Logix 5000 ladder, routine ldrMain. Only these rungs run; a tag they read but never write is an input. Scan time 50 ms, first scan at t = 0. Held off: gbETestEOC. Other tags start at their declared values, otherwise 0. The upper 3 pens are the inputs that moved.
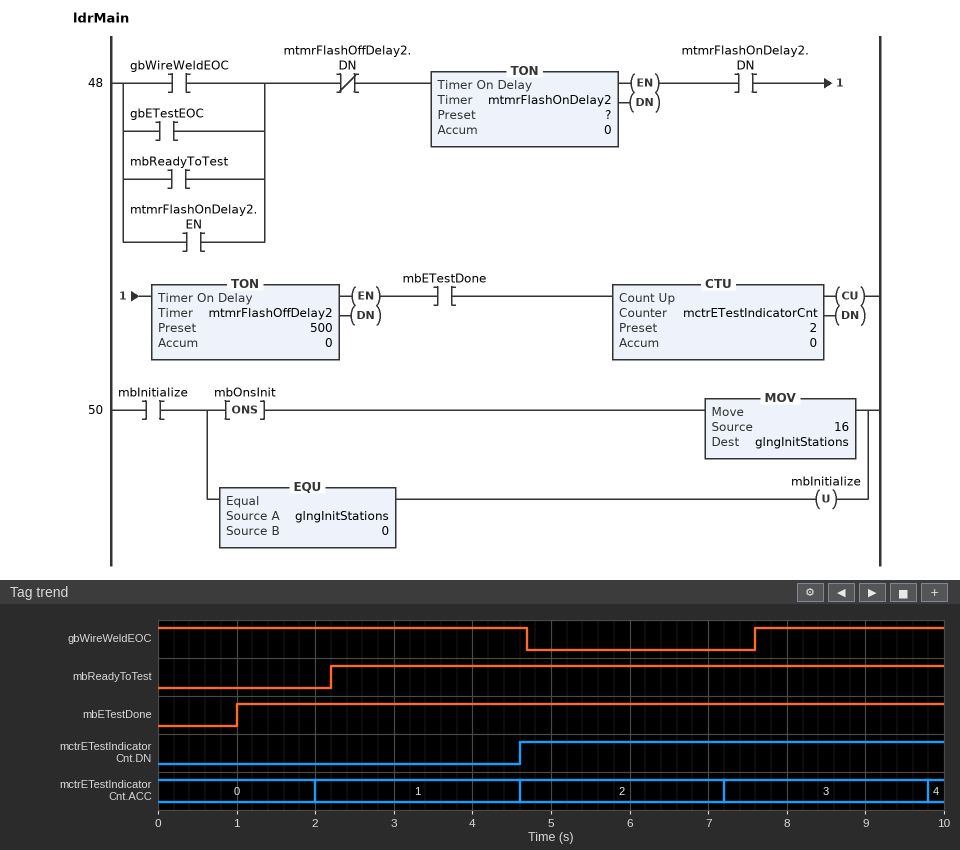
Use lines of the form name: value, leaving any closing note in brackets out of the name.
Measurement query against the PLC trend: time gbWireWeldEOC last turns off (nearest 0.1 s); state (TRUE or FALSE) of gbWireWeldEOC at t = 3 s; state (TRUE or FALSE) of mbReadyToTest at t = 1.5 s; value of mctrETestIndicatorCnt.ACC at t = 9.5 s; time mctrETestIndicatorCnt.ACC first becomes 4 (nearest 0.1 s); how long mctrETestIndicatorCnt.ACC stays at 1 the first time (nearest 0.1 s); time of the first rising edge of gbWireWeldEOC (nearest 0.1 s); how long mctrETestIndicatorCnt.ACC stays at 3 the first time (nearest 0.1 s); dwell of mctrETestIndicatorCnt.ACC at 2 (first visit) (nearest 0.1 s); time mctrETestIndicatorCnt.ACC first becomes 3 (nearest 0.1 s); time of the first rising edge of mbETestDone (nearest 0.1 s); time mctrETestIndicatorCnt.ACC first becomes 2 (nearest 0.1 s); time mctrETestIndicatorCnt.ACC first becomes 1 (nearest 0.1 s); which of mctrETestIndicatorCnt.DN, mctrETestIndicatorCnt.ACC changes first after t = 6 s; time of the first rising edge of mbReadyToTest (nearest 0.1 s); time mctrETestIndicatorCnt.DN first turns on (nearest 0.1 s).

time gbWireWeldEOC last turns off: 4.7 s
state (TRUE or FALSE) of gbWireWeldEOC at t = 3 s: TRUE
state (TRUE or FALSE) of mbReadyToTest at t = 1.5 s: FALSE
value of mctrETestIndicatorCnt.ACC at t = 9.5 s: 3
time mctrETestIndicatorCnt.ACC first becomes 4: 9.8 s
how long mctrETestIndicatorCnt.ACC stays at 1 the first time: 2.6 s
time of the first rising edge of gbWireWeldEOC: 7.6 s
how long mctrETestIndicatorCnt.ACC stays at 3 the first time: 2.6 s
dwell of mctrETestIndicatorCnt.ACC at 2 (first visit): 2.6 s
time mctrETestIndicatorCnt.ACC first becomes 3: 7.2 s
time of the first rising edge of mbETestDone: 1.0 s
time mctrETestIndicatorCnt.ACC first becomes 2: 4.6 s
time mctrETestIndicatorCnt.ACC first becomes 1: 2.0 s
which of mctrETestIndicatorCnt.DN, mctrETestIndicatorCnt.ACC changes first after t = 6 s: mctrETestIndicatorCnt.ACC
time of the first rising edge of mbReadyToTest: 2.2 s
time mctrETestIndicatorCnt.DN first turns on: 4.6 s
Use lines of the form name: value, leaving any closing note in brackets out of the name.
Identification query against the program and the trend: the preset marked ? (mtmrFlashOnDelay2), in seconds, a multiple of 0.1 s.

the preset marked ? (mtmrFlashOnDelay2), in seconds, a multiple of 0.1 s: 2.0 s
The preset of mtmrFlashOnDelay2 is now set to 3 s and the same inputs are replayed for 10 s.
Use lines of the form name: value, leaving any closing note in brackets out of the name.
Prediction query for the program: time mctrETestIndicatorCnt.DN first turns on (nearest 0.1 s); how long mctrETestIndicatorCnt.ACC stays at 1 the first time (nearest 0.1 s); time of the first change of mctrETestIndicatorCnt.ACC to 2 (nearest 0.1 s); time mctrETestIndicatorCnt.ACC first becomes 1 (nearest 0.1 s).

time mctrETestIndicatorCnt.DN first turns on: 6.6 s
how long mctrETestIndicatorCnt.ACC stays at 1 the first time: 3.6 s
time of the first change of mctrETestIndicatorCnt.ACC to 2: 6.6 s
time mctrETestIndicatorCnt.ACC first becomes 1: 3.0 s
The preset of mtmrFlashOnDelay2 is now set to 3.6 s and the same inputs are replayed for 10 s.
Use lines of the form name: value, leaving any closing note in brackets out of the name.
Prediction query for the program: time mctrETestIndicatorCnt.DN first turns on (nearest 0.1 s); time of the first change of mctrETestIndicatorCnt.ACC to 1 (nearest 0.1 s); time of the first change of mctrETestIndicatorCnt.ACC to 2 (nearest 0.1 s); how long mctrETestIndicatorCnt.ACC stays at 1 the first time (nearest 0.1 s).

time mctrETestIndicatorCnt.DN first turns on: 7.8 s
time of the first change of mctrETestIndicatorCnt.ACC to 1: 3.6 s
time of the first change of mctrETestIndicatorCnt.ACC to 2: 7.8 s
how long mctrETestIndicatorCnt.ACC stays at 1 the first time: 4.2 s
